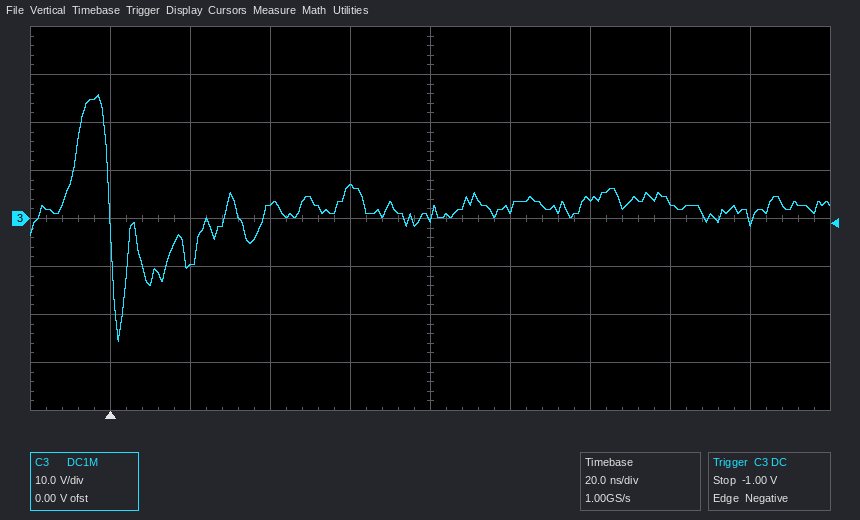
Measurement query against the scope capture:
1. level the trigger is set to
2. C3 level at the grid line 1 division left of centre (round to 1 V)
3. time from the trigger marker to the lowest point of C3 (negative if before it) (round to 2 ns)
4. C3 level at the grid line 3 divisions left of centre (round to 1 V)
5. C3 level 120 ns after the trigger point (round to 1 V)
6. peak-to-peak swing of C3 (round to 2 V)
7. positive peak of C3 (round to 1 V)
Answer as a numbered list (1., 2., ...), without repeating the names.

1. -1.00 V
2. 7 V
3. +2 ns
4. -10 V
5. 4 V
6. 52 V
7. 26 V
